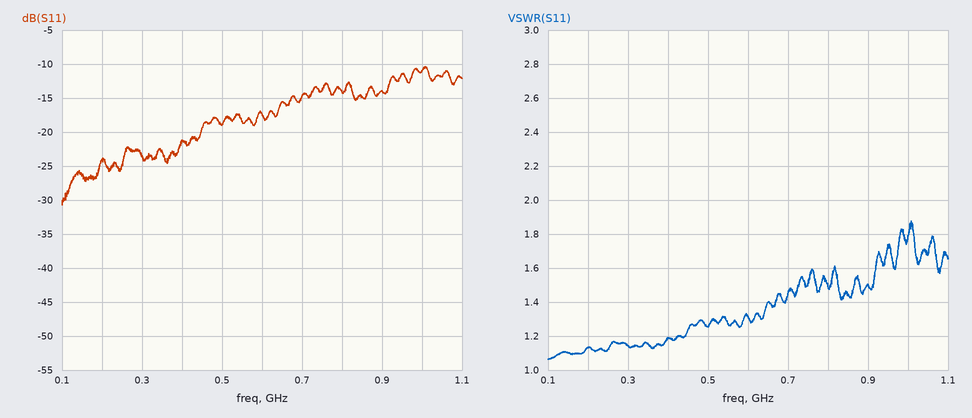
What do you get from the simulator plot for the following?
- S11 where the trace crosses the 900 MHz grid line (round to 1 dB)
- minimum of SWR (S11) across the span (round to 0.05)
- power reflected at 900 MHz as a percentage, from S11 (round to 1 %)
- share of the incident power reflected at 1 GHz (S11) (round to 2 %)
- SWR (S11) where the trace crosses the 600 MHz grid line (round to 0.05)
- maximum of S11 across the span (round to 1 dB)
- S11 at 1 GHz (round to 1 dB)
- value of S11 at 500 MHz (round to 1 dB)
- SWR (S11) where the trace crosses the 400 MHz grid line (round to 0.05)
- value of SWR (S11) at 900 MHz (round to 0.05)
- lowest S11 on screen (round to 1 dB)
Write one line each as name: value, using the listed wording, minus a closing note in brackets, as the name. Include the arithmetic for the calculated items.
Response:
S11 where the trace crosses the 900 MHz grid line: -14 dB
minimum of SWR (S11) across the span: 1.05
power reflected at 900 MHz as a percentage, from S11: 10^(-14/10) ≈ 4 %
share of the incident power reflected at 1 GHz (S11): 10^(-11/10) ≈ 8 %
SWR (S11) where the trace crosses the 600 MHz grid line: 1.30
maximum of S11 across the span: -10 dB
S11 at 1 GHz: -11 dB
value of S11 at 500 MHz: -19 dB
SWR (S11) where the trace crosses the 400 MHz grid line: 1.20
value of SWR (S11) at 900 MHz: 1.50
lowest S11 on screen: -31 dB
